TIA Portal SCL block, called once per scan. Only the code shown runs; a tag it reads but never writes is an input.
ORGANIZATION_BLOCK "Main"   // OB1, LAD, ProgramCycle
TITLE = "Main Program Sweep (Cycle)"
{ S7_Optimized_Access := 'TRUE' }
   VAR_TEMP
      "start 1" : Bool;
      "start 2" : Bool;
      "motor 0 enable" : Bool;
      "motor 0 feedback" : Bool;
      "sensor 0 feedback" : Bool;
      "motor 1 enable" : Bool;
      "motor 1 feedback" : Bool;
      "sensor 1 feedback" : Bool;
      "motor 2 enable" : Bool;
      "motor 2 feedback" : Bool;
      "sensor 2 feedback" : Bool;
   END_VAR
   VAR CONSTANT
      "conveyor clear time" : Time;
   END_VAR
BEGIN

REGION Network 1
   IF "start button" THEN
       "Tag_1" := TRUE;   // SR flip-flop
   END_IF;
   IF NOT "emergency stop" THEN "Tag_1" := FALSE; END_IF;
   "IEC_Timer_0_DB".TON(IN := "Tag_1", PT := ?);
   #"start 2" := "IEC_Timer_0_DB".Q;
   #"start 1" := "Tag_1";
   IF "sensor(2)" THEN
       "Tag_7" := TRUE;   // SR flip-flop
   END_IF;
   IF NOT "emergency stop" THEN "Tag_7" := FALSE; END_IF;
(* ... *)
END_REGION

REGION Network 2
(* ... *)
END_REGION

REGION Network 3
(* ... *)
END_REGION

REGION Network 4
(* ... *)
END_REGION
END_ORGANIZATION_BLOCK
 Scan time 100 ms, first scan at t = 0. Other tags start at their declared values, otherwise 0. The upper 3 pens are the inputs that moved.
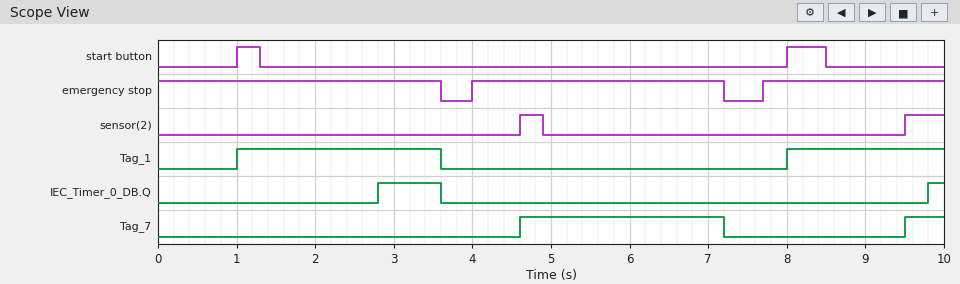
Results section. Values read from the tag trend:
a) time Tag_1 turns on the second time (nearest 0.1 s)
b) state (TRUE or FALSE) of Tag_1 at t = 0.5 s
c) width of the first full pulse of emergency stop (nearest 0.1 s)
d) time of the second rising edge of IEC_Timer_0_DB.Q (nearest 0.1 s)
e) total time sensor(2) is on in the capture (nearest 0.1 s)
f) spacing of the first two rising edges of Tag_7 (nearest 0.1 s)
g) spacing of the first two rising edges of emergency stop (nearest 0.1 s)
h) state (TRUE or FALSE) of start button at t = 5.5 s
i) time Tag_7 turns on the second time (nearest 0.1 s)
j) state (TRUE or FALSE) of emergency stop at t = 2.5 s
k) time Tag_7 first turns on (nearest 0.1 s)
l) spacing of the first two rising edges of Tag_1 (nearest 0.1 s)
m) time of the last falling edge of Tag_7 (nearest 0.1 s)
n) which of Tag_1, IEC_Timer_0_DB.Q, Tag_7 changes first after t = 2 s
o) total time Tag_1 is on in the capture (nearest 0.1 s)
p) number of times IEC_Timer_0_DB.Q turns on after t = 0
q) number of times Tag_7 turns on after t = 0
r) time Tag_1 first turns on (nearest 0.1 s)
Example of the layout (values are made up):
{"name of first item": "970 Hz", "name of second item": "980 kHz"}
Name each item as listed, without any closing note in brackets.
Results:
{"time Tag_1 turns on the second time": "8.0 s", "state (TRUE or FALSE) of Tag_1 at t = 0.5 s": "FALSE", "width of the first full pulse of emergency stop": "3.2 s", "time of the second rising edge of IEC_Timer_0_DB.Q": "9.8 s", "total time sensor(2) is on in the capture": "0.8 s", "spacing of the first two rising edges of Tag_7": "4.9 s", "spacing of the first two rising edges of emergency stop": "3.7 s", "state (TRUE or FALSE) of start button at t = 5.5 s": "FALSE", "time Tag_7 turns on the second time": "9.5 s", "state (TRUE or FALSE) of emergency stop at t = 2.5 s": "TRUE", "time Tag_7 first turns on": "4.6 s", "spacing of the first two rising edges of Tag_1": "7.0 s", "time of the last falling edge of Tag_7": "7.2 s", "which of Tag_1, IEC_Timer_0_DB.Q, Tag_7 changes first after t = 2 s": "IEC_Timer_0_DB.Q", "total time Tag_1 is on in the capture": "4.6 s", "number of times IEC_Timer_0_DB.Q turns on after t = 0": "2", "number of times Tag_7 turns on after t = 0": "2", "time Tag_1 first turns on": "1.0 s"}
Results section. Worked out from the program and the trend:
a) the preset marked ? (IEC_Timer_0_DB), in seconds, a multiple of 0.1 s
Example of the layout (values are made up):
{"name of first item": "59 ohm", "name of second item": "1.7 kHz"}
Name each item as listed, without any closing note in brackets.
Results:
{"the preset marked ? (IEC_Timer_0_DB), in seconds, a multiple of 0.1 s": "1.8 s"}
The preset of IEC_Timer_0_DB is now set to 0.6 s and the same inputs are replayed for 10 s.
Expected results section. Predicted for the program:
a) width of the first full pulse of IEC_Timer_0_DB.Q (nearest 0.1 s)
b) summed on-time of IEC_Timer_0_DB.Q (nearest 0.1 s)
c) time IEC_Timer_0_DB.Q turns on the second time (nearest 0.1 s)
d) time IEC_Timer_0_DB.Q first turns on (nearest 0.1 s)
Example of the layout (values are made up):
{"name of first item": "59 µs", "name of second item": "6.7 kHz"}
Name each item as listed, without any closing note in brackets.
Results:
{"width of the first full pulse of IEC_Timer_0_DB.Q": "2.0 s", "summed on-time of IEC_Timer_0_DB.Q": "3.4 s", "time IEC_Timer_0_DB.Q turns on the second time": "8.6 s", "time IEC_Timer_0_DB.Q first turns on": "1.6 s"}
